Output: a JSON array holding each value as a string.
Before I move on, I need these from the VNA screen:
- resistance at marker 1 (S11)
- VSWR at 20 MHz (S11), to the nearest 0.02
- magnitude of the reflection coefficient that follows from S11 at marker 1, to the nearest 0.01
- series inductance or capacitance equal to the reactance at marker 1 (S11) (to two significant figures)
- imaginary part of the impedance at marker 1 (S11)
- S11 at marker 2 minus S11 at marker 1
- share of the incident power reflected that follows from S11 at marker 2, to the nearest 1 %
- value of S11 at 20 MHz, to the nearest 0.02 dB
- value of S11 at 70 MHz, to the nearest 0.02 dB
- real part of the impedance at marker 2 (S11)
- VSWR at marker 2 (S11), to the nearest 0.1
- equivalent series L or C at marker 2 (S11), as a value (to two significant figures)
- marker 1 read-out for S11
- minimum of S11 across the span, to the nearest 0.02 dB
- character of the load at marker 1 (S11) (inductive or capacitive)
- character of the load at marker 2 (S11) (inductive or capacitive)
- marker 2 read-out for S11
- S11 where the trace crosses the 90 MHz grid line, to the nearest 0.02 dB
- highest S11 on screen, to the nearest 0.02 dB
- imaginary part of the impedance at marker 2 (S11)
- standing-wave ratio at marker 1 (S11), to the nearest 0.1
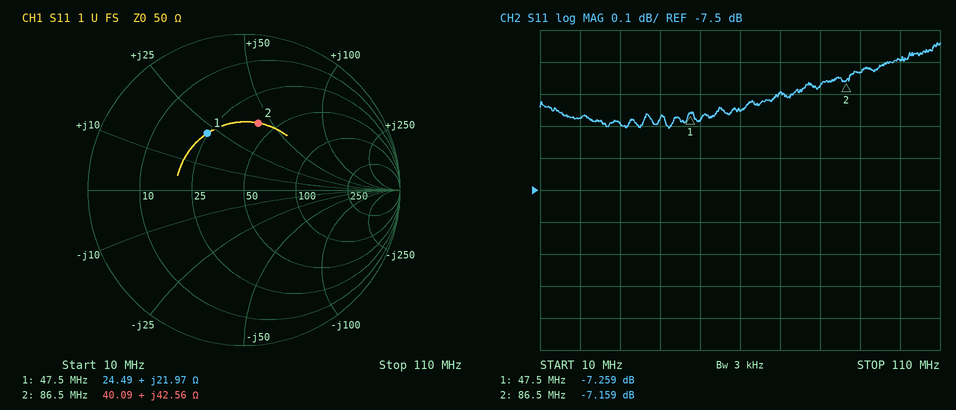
["24.49 Ω", "2.52", "0.43", "74 nH", "+21.97 Ω", "0.100 dB", "19 %", "-7.28 dB", "-7.20 dB", "40.09 Ω", "2.6", "78 nH", "-7.259 dB", "-7.30 dB", "inductive", "inductive", "-7.159 dB", "-7.14 dB", "-7.04 dB", "+42.56 Ω", "2.5"]
